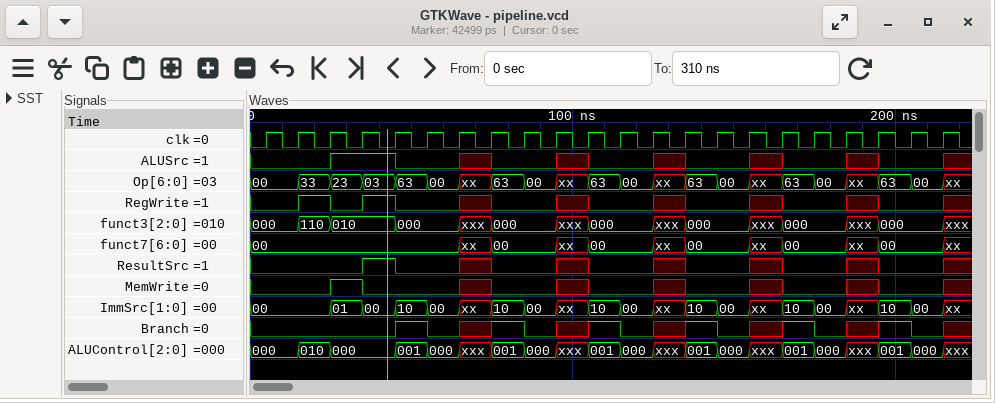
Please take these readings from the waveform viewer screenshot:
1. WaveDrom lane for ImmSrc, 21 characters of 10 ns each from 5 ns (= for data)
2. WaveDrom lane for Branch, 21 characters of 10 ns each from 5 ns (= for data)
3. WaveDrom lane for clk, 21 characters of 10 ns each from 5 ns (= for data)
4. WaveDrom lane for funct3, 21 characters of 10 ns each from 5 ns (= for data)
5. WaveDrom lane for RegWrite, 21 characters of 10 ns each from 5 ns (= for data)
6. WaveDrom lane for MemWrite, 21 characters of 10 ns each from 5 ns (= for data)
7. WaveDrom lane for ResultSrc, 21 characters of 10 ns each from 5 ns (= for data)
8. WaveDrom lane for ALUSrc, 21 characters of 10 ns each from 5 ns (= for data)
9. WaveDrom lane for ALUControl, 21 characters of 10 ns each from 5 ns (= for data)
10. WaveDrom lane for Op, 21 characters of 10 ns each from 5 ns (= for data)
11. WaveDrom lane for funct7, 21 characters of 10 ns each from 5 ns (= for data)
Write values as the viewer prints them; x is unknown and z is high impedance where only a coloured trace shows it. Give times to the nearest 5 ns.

{name: 'ImmSrc', wave: '=.====x==x==x==x==x==', data: '00 01 00 10 00 10 00 10 00 10 00 10 00 10 00'}
{name: 'Branch', wave: '0...10x10x10x10x10x10'}
{name: 'clk', wave: 'p....................'}
{name: 'funct3', wave: '===.=.x=.x=.x=.x=.x=.', data: '000 110 010 000 000 000 000 000 000'}
{name: 'RegWrite', wave: '01010.x0.x0.x0.x0.x0.'}
{name: 'MemWrite', wave: '0.10..x0.x0.x0.x0.x0.'}
{name: 'ResultSrc', wave: '0..10.x0.x0.x0.x0.x0.'}
{name: 'ALUSrc', wave: '0.1.0.x0.x0.x0.x0.x0.'}
{name: 'ALUControl', wave: '===.==x==x==x==x==x==', data: '000 010 000 001 000 001 000 001 000 001 000 001 000 001 000'}
{name: 'Op', wave: '======x==x==x==x==x==', data: '00 33 23 03 63 00 63 00 63 00 63 00 63 00 63 00'}
{name: 'funct7', wave: '=.....x=.x=.x=.x=.x=.', data: '00 00 00 00 00 00'}
